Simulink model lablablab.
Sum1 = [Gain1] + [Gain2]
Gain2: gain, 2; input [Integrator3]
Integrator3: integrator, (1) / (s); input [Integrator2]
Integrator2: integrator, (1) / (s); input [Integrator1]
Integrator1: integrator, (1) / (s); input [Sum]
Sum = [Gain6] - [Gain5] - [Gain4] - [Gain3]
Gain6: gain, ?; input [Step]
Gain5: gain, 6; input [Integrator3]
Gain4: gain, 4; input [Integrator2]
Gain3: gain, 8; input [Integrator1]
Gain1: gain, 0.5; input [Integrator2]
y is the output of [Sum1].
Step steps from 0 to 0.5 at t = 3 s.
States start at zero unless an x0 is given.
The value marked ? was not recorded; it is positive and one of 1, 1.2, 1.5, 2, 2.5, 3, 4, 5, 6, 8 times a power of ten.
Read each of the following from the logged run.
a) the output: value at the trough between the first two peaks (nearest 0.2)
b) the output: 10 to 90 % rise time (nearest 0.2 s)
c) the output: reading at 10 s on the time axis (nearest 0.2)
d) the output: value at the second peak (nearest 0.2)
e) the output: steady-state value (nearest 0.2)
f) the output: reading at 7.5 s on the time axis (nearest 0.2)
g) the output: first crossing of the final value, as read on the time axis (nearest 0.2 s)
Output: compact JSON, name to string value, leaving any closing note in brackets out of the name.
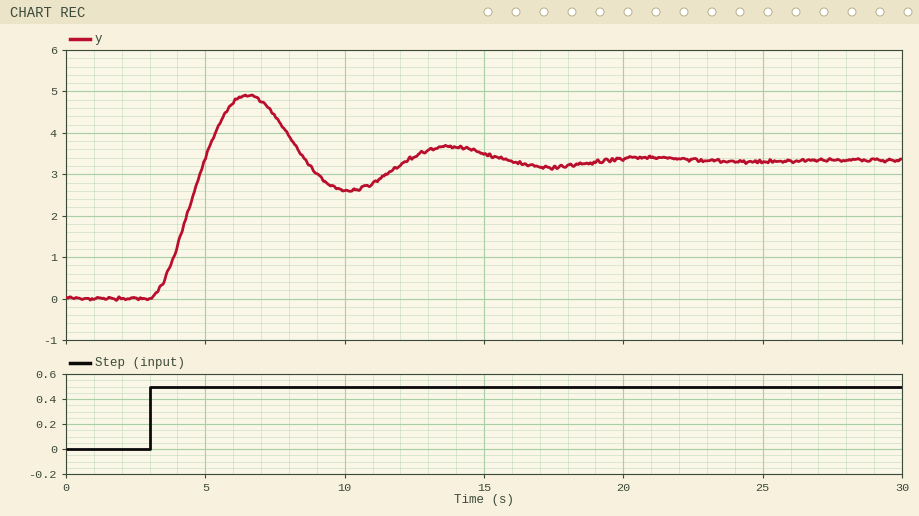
{"the output: value at the trough between the first two peaks": "2.6", "the output: 10 to 90 % rise time": "1.4 s", "the output: reading at 10 s on the time axis": "2.6", "the output: value at the second peak": "3.6", "the output: steady-state value": "3.4", "the output: reading at 7.5 s on the time axis": "4.4", "the output: first crossing of the final value, as read on the time axis": "5.0 s"}
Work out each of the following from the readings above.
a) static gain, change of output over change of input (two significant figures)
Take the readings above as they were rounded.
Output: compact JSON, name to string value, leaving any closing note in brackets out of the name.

{"static gain, change of output over change of input": "6.8"}
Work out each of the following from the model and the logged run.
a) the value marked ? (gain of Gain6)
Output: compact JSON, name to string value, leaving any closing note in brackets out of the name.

{"the value marked ?": "20"}
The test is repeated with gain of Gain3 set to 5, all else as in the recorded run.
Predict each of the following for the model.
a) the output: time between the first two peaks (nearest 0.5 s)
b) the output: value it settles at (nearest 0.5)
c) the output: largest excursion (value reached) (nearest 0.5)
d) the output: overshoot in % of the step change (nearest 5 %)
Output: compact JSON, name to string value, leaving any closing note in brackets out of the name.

{"the output: time between the first two peaks": "5.5 s", "the output: value it settles at": "3.5", "the output: largest excursion (value reached)": "5.0", "the output: overshoot in % of the step change": "45 %"}
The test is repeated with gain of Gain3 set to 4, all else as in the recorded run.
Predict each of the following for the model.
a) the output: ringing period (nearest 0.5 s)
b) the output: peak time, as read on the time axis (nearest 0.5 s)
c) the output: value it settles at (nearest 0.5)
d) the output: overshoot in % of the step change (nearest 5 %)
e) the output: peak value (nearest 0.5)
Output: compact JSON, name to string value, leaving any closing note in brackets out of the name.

{"the output: ringing period": "5.0 s", "the output: peak time, as read on the time axis": "5.5 s", "the output: value it settles at": "3.5", "the output: overshoot in % of the step change": "45 %", "the output: peak value": "5.0"}
